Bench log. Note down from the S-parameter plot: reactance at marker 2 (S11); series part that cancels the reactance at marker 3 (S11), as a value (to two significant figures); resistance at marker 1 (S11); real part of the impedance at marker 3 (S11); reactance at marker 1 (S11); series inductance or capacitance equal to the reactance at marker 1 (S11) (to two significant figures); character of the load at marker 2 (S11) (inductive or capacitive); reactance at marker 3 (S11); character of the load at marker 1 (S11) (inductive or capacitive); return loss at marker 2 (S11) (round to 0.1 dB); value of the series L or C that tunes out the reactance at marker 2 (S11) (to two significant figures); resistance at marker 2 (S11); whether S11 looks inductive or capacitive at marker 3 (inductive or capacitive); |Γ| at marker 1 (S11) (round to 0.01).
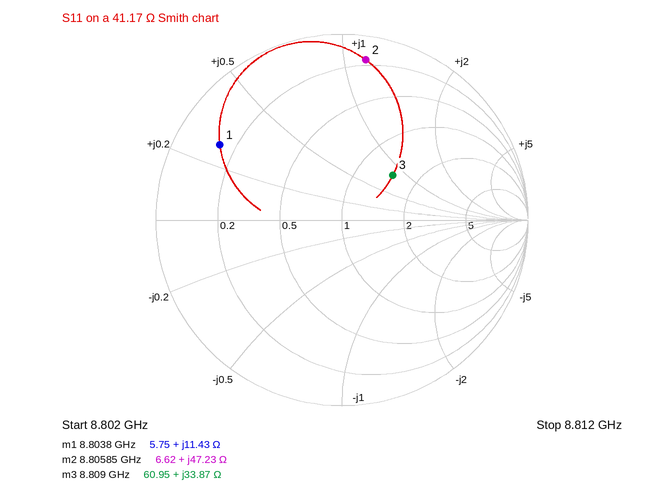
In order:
+47.23 Ω
530 fF
5.75 Ω
60.95 Ω
+11.43 Ω
210 pH
inductive
+33.87 Ω
inductive
1.2 dB
380 fF
6.62 Ω
inductive
0.77
